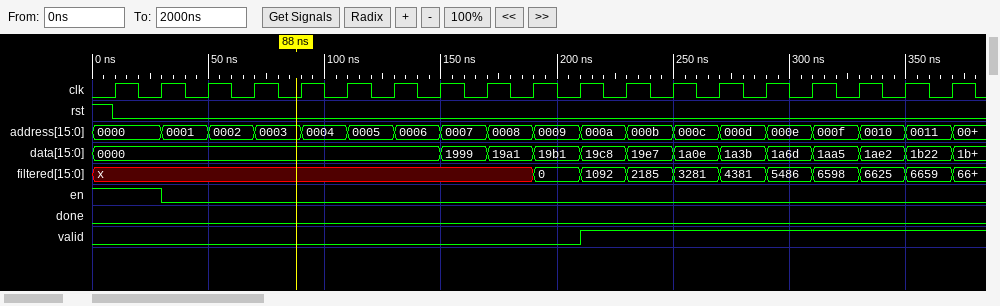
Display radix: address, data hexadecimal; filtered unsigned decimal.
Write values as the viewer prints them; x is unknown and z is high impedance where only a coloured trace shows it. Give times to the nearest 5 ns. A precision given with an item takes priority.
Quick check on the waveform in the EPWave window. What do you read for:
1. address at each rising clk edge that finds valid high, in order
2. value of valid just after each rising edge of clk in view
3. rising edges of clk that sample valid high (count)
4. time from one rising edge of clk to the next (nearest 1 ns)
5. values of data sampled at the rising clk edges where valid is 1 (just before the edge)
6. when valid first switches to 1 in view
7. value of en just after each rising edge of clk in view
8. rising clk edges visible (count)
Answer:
000a, 000b, 000c, 000d, 000e, 000f, 0010, 0011
0 0 0 0 0 0 0 0 0 0 1 1 1 1 1 1 1 1 1
8
20 ns
19c8, 19e7, 1a0e, 1a3b, 1a6d, 1aa5, 1ae2, 1b22
210 ns
1 0 0 0 0 0 0 0 0 0 0 0 0 0 0 0 0 0 0
19
